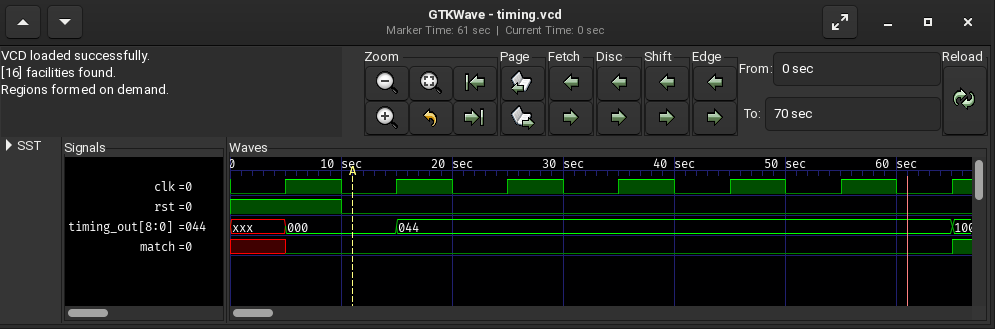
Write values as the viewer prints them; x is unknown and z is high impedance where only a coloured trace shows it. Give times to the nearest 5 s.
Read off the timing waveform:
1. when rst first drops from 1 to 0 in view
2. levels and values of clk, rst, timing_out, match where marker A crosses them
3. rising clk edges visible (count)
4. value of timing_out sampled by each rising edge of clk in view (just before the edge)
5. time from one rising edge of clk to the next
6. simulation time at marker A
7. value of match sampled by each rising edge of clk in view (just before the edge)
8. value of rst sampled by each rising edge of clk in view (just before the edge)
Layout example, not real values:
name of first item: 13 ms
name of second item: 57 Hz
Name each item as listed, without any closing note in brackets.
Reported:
when rst first drops from 1 to 0 in view: 10 s
levels and values of clk, rst, timing_out, match where marker A crosses them: clk=0, rst=0, timing_out=000, match=0
rising clk edges visible: 7
value of timing_out sampled by each rising edge of clk in view: xxx, 000, 044, 044, 044, 044, 044
time from one rising edge of clk to the next: 10 s
simulation time at marker A: 10 s
value of match sampled by each rising edge of clk in view: x 0 0 0 0 0 0
value of rst sampled by each rising edge of clk in view: 1 0 0 0 0 0 0
